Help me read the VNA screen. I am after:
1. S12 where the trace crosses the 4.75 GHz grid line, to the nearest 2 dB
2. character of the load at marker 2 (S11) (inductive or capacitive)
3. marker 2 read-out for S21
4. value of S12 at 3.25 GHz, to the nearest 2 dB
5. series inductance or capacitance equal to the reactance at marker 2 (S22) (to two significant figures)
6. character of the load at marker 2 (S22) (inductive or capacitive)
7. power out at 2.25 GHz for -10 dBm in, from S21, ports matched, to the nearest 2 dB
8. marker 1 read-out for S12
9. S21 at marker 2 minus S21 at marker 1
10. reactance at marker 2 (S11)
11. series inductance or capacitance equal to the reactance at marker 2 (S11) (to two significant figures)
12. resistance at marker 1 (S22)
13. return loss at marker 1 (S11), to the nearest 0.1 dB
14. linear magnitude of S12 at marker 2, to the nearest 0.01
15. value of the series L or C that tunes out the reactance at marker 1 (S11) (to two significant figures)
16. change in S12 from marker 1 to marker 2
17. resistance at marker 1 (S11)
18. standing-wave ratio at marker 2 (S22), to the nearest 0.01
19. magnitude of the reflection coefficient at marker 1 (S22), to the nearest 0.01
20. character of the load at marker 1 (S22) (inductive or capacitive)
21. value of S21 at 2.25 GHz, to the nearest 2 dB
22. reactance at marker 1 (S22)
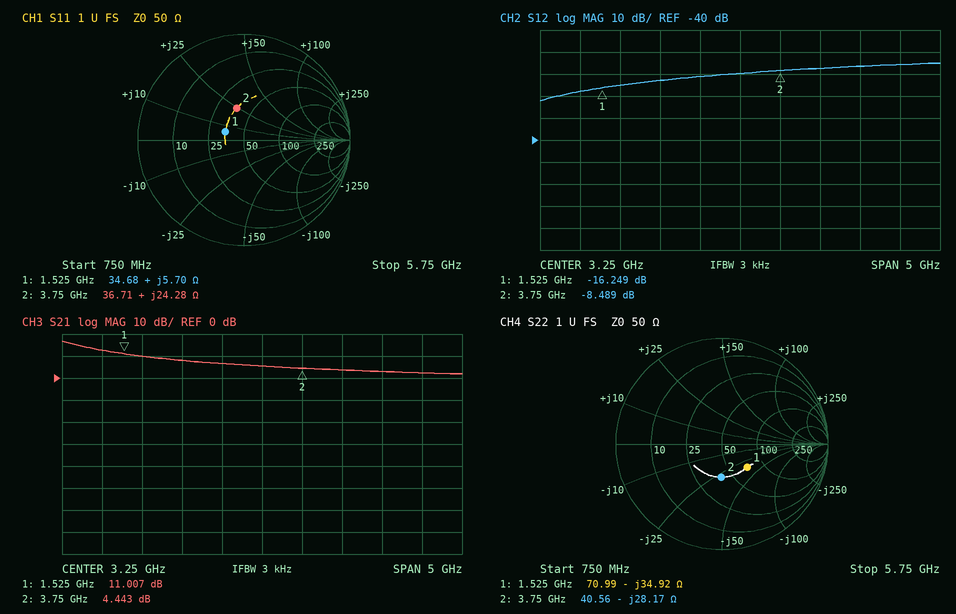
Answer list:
-6 dB
inductive
4.443 dB
-10 dB
1.5 pF
capacitive
-2 dBm
-16.249 dB
-6.564 dB
+24.28 Ω
1.0 nH
70.99 Ω
14.3 dB
0.38
18 pF
7.760 dB
34.68 Ω
1.91
0.32
capacitive
8 dB
-34.92 Ω
